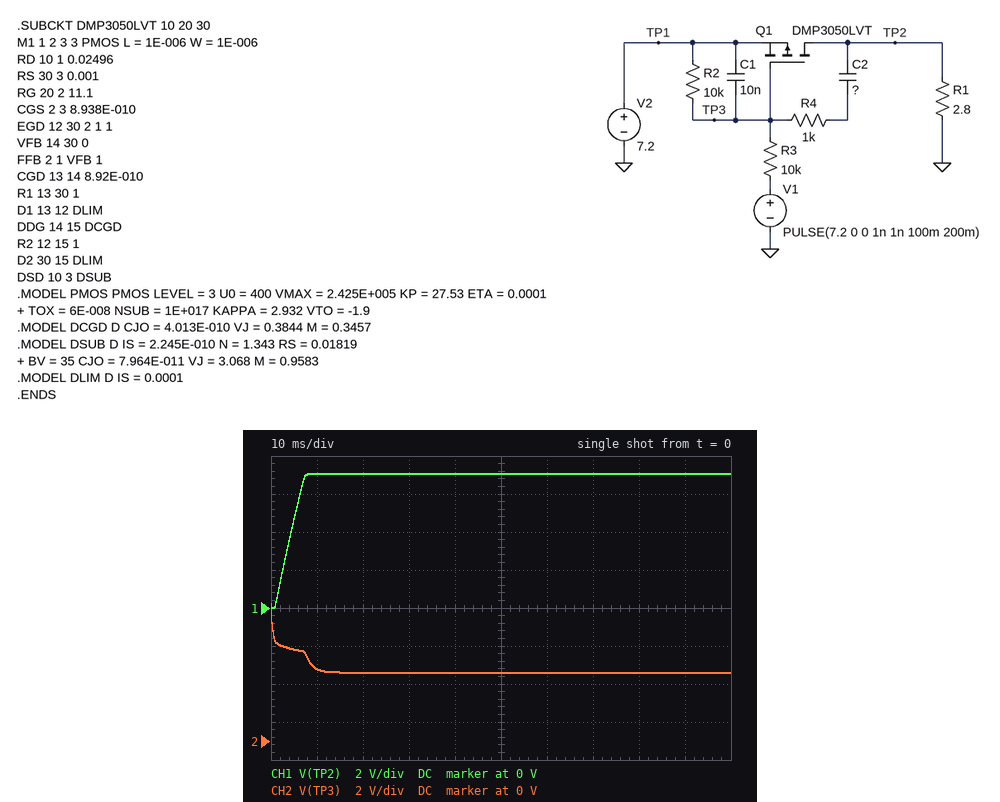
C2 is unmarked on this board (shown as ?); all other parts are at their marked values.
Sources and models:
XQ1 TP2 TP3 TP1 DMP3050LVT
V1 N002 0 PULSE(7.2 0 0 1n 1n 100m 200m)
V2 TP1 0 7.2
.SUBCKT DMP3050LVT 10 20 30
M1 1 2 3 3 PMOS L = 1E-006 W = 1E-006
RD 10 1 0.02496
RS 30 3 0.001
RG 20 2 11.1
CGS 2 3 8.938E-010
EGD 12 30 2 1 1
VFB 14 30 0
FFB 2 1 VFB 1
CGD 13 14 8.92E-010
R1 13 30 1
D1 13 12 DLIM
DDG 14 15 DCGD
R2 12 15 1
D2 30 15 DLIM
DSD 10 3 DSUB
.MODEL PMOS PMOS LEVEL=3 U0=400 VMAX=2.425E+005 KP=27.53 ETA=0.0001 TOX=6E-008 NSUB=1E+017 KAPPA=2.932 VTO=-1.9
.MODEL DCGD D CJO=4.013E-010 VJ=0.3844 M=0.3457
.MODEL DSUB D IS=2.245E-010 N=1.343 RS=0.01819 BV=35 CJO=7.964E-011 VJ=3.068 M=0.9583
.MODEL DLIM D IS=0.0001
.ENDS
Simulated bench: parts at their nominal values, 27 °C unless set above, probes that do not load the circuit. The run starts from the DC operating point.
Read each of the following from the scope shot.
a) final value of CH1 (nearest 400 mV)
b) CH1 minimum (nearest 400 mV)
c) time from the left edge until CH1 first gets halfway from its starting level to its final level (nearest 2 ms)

7.2 V
0 V
4 ms
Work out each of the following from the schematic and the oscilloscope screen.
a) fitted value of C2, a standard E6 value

220 nF
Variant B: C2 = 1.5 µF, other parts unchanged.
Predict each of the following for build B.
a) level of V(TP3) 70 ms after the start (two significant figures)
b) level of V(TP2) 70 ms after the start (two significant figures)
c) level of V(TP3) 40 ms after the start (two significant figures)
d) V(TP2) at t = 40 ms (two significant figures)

3.7 V
7.1 V
4.8 V
5.6 V
